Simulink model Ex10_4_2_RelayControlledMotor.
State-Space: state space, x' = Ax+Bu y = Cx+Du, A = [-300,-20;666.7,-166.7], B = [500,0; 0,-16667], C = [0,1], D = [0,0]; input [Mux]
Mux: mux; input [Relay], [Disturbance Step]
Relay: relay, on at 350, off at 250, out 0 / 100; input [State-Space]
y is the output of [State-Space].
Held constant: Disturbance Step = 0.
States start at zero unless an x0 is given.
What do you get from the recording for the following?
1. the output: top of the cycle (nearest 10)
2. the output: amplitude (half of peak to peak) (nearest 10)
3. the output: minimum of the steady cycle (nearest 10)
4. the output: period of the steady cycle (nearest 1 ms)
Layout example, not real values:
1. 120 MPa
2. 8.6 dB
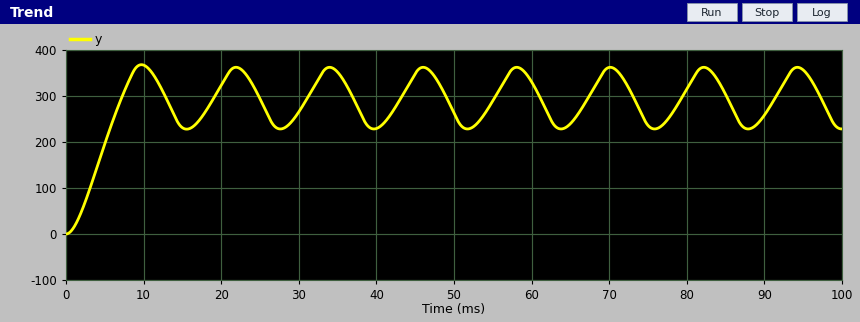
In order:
1. 360
2. 70
3. 230
4. 12 ms
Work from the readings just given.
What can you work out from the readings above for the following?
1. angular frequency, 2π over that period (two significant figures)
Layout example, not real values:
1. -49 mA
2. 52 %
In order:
1. 0.52 rad/ms
